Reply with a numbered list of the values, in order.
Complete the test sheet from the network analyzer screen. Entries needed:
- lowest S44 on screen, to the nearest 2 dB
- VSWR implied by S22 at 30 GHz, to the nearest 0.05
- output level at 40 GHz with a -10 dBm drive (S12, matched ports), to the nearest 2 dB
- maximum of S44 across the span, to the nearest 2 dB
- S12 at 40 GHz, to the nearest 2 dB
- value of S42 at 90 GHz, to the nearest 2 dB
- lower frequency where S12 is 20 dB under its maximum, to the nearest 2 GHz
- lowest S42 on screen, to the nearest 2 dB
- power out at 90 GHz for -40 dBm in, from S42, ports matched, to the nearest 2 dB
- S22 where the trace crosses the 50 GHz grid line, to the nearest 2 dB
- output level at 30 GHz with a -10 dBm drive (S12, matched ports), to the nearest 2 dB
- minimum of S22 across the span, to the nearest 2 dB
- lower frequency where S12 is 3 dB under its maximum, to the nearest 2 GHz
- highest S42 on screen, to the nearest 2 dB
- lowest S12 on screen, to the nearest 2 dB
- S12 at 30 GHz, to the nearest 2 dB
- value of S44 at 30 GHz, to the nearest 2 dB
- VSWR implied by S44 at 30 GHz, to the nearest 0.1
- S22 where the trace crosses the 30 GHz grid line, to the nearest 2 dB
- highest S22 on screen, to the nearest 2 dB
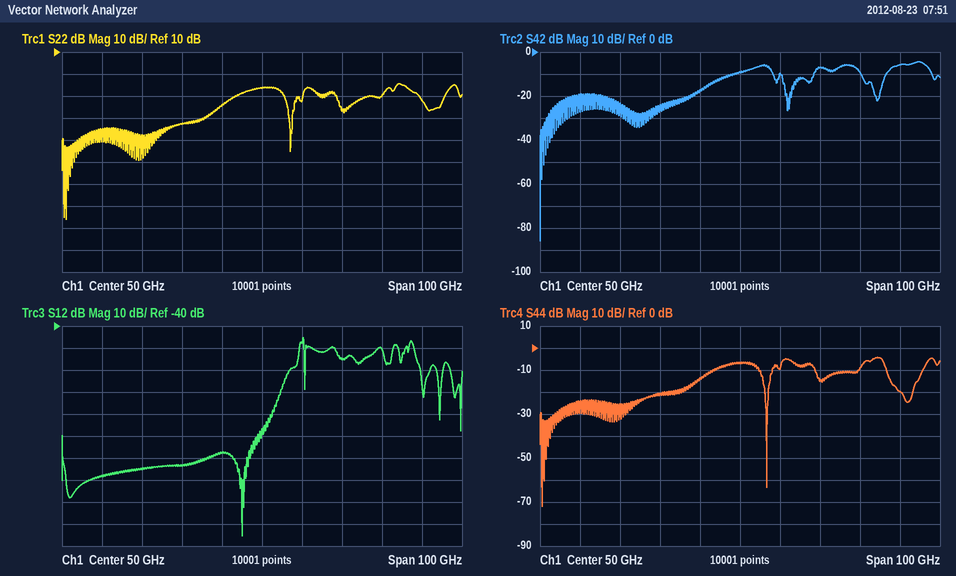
1. -72 dB
2. 1.15
3. -108 dBm
4. -4 dB
5. -98 dB
6. -6 dB
7. 56 GHz
8. -86 dB
9. -46 dBm
10. -6 dB
11. -114 dBm
12. -66 dB
13. 60 GHz
14. -4 dB
15. -136 dB
16. -104 dB
17. -20 dB
18. 1.2
19. -22 dB
20. -4 dB
